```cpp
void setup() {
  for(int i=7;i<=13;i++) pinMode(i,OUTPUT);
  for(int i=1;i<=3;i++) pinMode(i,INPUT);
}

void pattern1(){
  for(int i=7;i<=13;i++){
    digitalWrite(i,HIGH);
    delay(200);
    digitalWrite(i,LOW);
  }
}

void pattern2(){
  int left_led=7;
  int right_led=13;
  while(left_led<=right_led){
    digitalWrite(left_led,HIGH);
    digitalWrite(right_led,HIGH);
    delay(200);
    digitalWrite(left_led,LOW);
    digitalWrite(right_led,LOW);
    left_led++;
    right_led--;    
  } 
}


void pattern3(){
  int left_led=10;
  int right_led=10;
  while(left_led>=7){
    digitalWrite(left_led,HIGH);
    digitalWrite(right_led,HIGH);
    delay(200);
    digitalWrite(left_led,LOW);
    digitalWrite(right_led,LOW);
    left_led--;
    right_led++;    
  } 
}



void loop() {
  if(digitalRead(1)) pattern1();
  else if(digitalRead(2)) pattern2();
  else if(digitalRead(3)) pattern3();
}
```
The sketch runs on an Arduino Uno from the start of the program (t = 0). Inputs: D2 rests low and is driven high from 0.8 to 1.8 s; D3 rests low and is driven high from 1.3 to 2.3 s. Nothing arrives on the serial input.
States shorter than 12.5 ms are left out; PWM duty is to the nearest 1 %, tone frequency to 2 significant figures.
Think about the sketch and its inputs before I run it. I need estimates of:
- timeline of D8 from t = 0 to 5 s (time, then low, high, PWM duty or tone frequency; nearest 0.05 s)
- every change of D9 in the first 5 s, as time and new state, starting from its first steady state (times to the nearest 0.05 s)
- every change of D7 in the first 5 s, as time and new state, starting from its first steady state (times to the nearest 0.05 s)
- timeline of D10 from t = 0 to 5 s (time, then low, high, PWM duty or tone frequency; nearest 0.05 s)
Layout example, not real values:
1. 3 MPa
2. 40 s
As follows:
1. 0 s low; 1 s high; 1.2 s low; 1.8 s high; 2 s low
2. 0 s low; 1.2 s high; 1.4 s low; 2 s high; 2.2 s low
3. 0 s low; 0.8 s high; 1 s low; 1.6 s high; 1.8 s low
4. 0 s low; 1.4 s high; 1.6 s low; 2.2 s high; 2.4 s low
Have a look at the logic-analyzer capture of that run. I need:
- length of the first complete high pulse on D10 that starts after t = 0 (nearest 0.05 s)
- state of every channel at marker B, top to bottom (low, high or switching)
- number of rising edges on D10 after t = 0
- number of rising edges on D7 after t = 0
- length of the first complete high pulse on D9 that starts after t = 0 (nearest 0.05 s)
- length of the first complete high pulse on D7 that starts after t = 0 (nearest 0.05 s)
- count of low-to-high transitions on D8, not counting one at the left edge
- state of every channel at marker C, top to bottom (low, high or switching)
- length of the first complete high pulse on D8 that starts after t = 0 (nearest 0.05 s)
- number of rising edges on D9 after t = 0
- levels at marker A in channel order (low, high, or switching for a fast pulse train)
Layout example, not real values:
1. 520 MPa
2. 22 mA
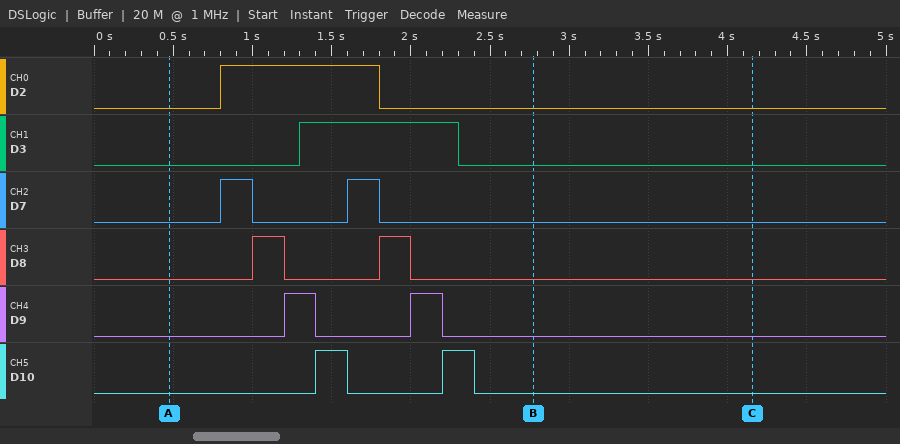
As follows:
1. 0.20 s
2. D2 low, D3 low, D7 low, D8 low, D9 low, D10 low
3. 2
4. 2
5. 0.20 s
6. 0.20 s
7. 2
8. D2 low, D3 low, D7 low, D8 low, D9 low, D10 low
9. 0.20 s
10. 2
11. D2 low, D3 low, D7 low, D8 low, D9 low, D10 low
